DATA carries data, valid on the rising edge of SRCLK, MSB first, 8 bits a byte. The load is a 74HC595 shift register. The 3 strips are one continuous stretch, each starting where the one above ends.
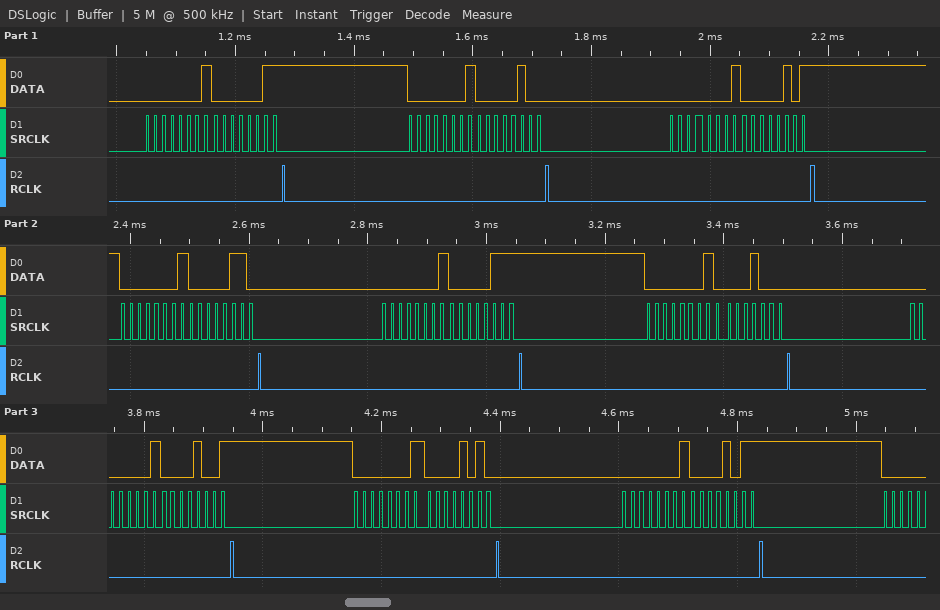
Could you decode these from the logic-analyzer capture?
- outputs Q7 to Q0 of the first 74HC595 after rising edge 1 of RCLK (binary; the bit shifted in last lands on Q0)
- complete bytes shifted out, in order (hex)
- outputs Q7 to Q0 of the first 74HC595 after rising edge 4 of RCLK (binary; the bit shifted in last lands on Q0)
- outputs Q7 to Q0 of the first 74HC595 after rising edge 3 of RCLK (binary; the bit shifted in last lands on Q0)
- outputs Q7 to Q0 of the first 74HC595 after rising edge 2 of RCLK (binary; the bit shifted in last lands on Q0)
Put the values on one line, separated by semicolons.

00000011; 01 03 01 04 01 05 01 06 01 07 01 08 01 09 01 0A 01 0B; 00000110; 00000101; 00000100
